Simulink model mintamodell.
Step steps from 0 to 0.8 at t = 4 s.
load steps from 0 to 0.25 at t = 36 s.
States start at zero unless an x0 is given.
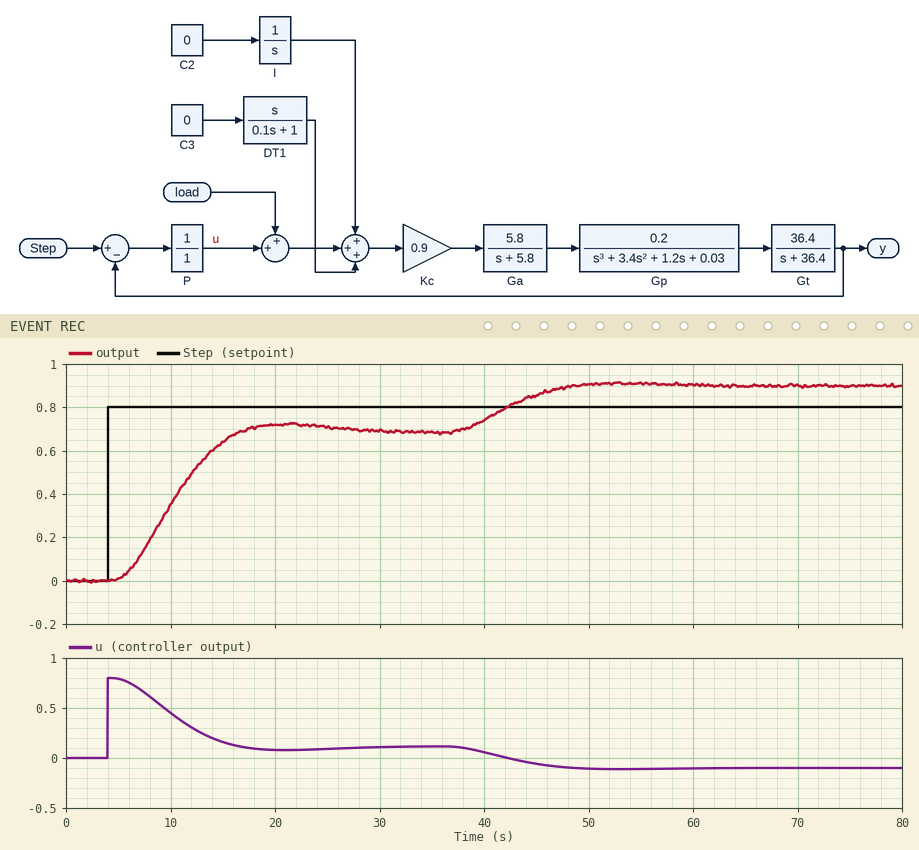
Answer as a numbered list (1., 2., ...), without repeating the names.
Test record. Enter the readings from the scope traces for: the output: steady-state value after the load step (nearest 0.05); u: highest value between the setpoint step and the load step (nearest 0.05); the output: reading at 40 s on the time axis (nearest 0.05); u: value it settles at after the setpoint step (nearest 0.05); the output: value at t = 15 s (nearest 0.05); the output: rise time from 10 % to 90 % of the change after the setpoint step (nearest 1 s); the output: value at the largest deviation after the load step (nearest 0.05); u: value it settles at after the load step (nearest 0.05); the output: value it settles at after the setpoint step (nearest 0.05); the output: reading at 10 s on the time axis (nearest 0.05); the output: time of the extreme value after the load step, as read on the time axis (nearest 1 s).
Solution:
1. 0.90
2. 0.80
3. 0.75
4. 0.10
5. 0.65
6. 8 s
7. 0.90
8. -0.10
9. 0.70
10. 0.35
11. 53 s
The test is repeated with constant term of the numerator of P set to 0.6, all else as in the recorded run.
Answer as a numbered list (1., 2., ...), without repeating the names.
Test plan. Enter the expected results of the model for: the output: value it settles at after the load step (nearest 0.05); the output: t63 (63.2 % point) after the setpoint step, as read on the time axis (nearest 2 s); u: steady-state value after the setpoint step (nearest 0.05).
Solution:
1. 0.95
2. 14 s
3. 0.10
